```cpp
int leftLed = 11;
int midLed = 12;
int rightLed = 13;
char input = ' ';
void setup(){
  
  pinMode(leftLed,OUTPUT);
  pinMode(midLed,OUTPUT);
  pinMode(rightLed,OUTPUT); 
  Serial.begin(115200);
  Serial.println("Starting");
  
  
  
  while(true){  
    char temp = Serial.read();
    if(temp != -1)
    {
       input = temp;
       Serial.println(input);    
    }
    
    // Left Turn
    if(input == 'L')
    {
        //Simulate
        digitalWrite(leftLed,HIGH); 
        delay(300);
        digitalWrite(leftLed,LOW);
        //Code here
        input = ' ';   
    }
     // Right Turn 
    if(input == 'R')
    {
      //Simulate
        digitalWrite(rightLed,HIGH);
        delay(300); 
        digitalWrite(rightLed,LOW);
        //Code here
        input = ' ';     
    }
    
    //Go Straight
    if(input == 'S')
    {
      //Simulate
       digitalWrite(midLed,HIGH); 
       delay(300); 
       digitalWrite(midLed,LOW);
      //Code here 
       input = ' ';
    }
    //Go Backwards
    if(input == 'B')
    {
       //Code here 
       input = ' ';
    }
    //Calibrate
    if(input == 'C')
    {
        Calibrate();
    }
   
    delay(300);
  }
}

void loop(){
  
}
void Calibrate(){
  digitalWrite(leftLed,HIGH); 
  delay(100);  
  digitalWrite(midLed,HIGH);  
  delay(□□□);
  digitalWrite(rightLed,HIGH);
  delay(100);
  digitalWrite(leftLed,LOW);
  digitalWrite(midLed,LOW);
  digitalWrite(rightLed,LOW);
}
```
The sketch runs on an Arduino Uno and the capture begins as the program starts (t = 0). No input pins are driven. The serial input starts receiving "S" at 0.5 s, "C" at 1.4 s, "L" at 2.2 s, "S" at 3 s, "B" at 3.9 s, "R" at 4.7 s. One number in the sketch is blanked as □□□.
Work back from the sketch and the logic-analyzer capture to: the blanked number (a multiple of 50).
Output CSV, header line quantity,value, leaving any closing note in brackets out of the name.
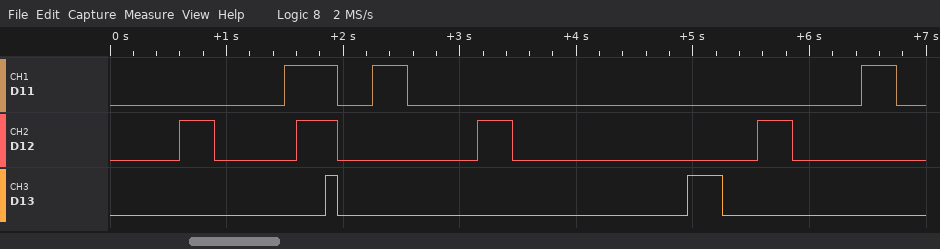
quantity,value
the blanked number,250
